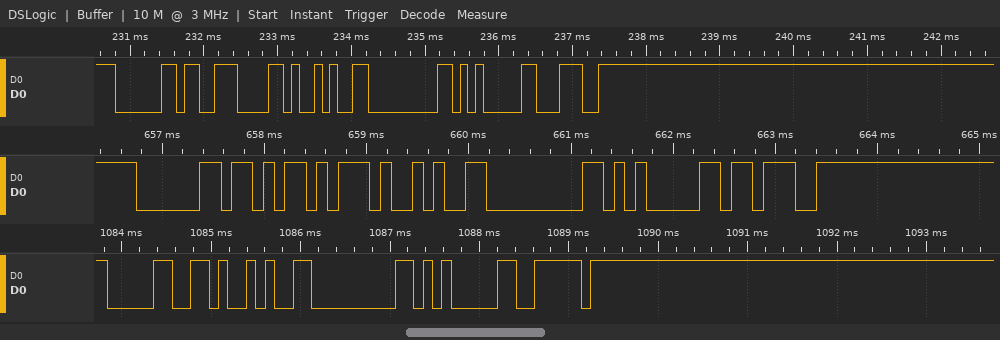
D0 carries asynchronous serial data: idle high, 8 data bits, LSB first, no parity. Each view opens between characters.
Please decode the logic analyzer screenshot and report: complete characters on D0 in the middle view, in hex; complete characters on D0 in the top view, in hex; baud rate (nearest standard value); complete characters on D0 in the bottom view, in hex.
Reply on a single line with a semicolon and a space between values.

60, AD, 29, 00, 05, 3B; 60, 0E, 29, 00, 05, 9C; 9600 baud; 30, 29, 00, 05, BE
